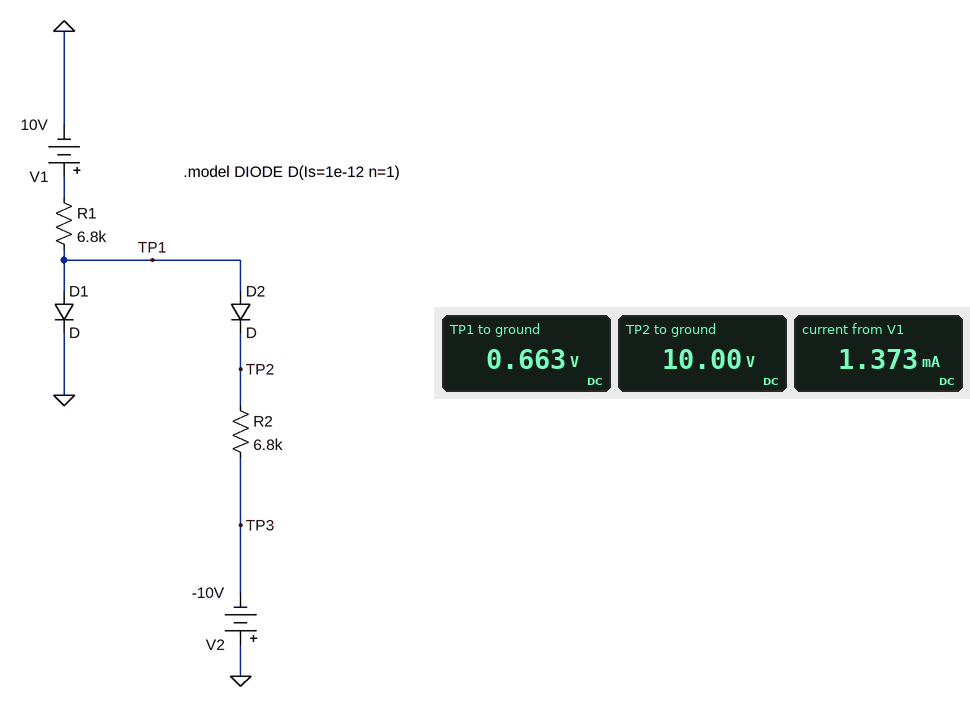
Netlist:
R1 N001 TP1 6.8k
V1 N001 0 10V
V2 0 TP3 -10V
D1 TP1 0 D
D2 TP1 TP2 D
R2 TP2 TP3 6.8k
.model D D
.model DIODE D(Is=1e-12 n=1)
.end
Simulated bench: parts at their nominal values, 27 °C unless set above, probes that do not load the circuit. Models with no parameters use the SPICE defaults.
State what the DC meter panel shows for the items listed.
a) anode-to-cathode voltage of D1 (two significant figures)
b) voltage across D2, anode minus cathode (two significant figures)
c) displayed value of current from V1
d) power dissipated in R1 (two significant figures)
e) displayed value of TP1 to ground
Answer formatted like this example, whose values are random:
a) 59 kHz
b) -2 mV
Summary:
a) 660 mV
b) -9.3 V
c) 1.373 mA
d) 13 mW
e) 0.663 V
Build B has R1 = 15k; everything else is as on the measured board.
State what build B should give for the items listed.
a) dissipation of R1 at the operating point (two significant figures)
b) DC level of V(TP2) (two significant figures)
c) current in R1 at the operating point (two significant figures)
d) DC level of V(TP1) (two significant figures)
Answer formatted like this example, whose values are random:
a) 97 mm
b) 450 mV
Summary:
a) 5.8 mW
b) 10 V
c) 620 µA
d) 640 mV
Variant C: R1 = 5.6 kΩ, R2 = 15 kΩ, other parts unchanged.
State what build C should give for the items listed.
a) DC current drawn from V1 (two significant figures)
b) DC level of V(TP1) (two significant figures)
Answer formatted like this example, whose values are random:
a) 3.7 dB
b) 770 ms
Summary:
a) 1.7 mA
b) 670 mV
